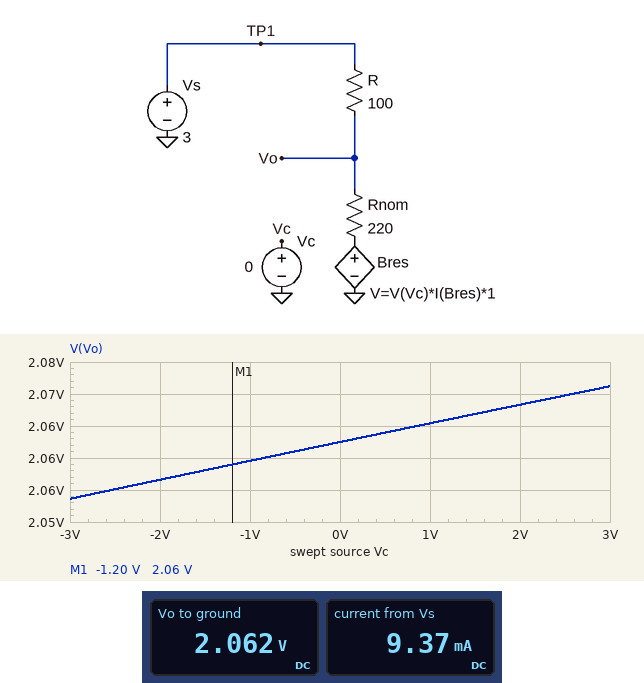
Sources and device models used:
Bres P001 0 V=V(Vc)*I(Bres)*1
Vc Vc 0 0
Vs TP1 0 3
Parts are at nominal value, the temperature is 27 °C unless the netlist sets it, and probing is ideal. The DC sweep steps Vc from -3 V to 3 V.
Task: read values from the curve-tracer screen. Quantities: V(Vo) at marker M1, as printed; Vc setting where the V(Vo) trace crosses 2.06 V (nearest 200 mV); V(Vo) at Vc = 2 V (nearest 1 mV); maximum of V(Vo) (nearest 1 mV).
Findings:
2.06 V
800 mV
2.068 V
2.071 V
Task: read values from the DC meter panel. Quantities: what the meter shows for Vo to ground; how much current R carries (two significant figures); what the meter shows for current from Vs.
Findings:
2.062 V
9.4 mA
9.37 mA
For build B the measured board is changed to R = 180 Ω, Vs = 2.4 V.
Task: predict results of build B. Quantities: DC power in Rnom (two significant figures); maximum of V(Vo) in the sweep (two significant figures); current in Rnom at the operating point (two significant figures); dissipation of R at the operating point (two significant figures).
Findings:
7.9 mW
1.3 V
6.0 mA
6.5 mW
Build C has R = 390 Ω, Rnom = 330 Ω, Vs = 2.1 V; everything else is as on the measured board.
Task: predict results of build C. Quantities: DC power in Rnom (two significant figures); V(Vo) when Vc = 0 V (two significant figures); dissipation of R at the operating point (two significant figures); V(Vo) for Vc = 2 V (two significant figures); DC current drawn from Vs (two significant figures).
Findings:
2.8 mW
960 mV
3.3 mW
970 mV
2.9 mA
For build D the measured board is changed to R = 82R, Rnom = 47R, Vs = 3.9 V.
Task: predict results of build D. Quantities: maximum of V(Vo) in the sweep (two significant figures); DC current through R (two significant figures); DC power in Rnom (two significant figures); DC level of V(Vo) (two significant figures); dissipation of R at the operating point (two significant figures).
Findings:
1.5 V
30 mA
43 mW
1.4 V
75 mW
